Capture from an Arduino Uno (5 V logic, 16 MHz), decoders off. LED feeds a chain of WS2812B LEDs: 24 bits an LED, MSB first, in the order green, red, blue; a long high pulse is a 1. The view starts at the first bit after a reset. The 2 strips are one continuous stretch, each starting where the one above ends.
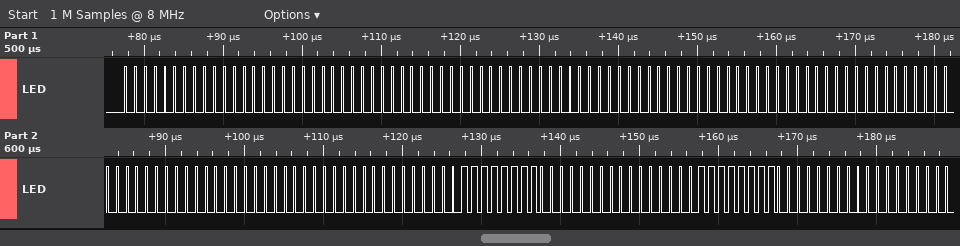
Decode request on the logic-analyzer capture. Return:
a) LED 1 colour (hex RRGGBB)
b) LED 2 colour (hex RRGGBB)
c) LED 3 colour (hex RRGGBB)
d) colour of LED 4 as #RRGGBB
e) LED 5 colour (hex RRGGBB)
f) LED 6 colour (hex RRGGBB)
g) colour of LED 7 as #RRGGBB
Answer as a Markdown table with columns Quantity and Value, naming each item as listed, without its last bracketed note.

| Quantity | Value |
|---|---|
| LED 1 colour | #000000 |
| LED 2 colour | #000000 |
| LED 3 colour | #000000 |
| colour of LED 4 as #RRGGBB | #000000 |
| LED 5 colour | #000000 |
| LED 6 colour | #00FF00 |
| colour of LED 7 as #RRGGBB | #00FF00 |
